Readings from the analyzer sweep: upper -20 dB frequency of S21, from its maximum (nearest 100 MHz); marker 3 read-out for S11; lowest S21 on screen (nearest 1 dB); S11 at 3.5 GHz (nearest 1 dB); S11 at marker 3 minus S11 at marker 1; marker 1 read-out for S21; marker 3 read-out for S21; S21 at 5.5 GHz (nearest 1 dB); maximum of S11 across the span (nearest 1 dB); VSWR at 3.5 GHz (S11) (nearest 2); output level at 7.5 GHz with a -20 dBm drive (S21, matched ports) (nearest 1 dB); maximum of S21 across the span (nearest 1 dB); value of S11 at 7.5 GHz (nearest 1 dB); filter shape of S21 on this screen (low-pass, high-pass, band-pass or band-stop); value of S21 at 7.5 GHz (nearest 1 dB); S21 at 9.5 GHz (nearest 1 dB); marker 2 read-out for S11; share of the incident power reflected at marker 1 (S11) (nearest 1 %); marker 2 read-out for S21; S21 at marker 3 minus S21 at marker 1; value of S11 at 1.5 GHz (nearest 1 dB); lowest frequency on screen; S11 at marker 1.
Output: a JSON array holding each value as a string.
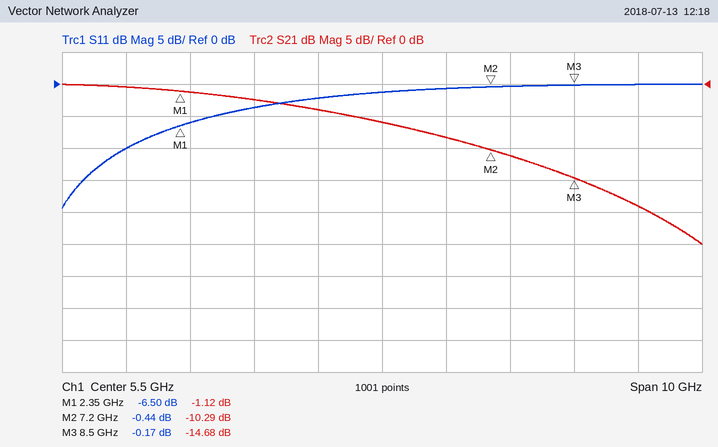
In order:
["9.7 GHz", "-0.17 dB", "-25 dB", "-4 dB", "6.33 dB", "-1.12 dB", "-14.68 dB", "-6 dB", "0 dB", "4", "-31 dBm", "0 dB", "0 dB", "low-pass", "-11 dB", "-19 dB", "-0.44 dB", "22 %", "-10.29 dB", "-13.56 dB", "-10 dB", "500 MHz", "-6.50 dB"]
